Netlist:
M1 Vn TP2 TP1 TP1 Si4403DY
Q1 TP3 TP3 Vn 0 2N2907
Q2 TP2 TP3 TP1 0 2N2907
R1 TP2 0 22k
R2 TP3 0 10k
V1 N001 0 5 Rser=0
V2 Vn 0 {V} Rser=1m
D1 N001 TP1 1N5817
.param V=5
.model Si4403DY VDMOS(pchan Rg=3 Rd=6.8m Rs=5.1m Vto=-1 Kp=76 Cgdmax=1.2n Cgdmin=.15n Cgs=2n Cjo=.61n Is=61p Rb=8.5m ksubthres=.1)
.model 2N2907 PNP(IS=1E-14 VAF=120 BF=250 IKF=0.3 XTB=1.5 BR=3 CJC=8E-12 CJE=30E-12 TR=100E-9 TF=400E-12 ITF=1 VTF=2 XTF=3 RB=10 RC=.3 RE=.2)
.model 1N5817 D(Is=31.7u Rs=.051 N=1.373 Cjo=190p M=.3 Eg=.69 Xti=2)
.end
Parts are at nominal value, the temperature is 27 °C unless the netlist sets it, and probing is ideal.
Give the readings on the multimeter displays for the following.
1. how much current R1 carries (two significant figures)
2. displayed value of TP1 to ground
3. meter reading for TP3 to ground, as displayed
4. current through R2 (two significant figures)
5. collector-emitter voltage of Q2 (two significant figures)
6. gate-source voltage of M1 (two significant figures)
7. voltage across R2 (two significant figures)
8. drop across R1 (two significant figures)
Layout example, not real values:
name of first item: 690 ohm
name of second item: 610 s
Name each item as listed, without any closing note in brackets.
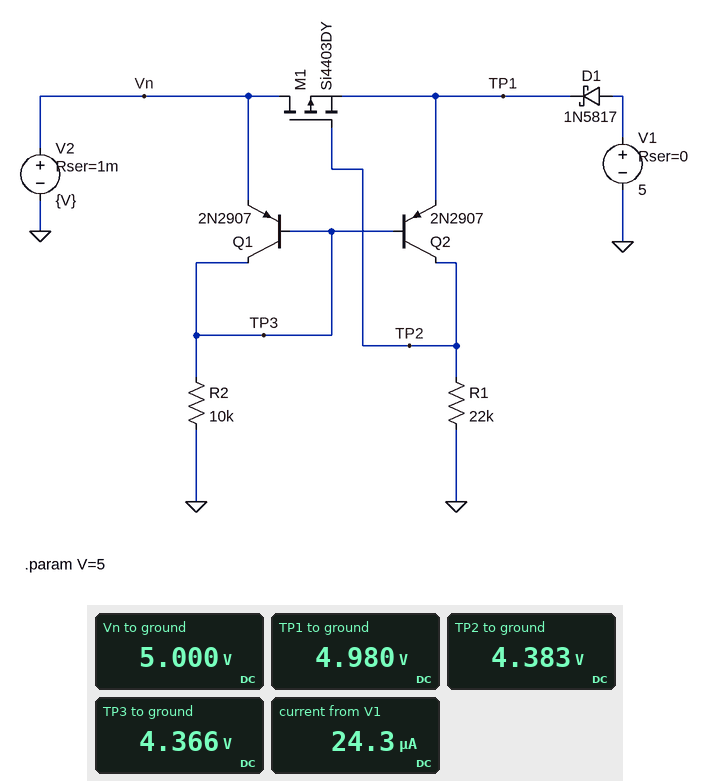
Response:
how much current R1 carries: 200 µA
displayed value of TP1 to ground: 4.980 V
meter reading for TP3 to ground, as displayed: 4.366 V
current through R2: 440 µA
collector-emitter voltage of Q2: -600 mV
gate-source voltage of M1: -600 mV
voltage across R2: 4.4 V
drop across R1: 4.4 V
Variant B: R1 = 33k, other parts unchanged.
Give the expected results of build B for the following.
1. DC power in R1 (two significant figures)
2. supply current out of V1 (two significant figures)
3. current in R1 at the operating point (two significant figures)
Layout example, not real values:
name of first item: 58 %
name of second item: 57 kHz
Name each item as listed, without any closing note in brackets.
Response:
DC power in R1: 590 µW
supply current out of V1: 43 µA
current in R1 at the operating point: 130 µA
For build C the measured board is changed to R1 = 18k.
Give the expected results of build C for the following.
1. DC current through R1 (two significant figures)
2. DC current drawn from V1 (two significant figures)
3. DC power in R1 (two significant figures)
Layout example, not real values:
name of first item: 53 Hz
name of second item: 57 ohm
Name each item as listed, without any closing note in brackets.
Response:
DC current through R1: 240 µA
DC current drawn from V1: 17 µA
DC power in R1: 1.1 mW
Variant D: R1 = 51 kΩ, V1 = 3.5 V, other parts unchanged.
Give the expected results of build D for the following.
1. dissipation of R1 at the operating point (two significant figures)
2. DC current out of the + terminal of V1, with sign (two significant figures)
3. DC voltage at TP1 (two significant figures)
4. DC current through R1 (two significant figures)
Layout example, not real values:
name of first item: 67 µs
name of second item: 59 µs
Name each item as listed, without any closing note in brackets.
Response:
dissipation of R1 at the operating point: 380 µW
DC current out of the + terminal of V1, with sign: -32 µA
DC voltage at TP1: 5.0 V
DC current through R1: 86 µA
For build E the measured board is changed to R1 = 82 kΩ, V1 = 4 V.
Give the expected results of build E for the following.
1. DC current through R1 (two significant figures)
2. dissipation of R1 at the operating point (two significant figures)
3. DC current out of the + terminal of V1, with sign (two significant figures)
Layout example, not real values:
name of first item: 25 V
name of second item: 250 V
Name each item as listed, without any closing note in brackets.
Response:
DC current through R1: 54 µA
dissipation of R1 at the operating point: 240 µW
DC current out of the + terminal of V1, with sign: -32 µA
